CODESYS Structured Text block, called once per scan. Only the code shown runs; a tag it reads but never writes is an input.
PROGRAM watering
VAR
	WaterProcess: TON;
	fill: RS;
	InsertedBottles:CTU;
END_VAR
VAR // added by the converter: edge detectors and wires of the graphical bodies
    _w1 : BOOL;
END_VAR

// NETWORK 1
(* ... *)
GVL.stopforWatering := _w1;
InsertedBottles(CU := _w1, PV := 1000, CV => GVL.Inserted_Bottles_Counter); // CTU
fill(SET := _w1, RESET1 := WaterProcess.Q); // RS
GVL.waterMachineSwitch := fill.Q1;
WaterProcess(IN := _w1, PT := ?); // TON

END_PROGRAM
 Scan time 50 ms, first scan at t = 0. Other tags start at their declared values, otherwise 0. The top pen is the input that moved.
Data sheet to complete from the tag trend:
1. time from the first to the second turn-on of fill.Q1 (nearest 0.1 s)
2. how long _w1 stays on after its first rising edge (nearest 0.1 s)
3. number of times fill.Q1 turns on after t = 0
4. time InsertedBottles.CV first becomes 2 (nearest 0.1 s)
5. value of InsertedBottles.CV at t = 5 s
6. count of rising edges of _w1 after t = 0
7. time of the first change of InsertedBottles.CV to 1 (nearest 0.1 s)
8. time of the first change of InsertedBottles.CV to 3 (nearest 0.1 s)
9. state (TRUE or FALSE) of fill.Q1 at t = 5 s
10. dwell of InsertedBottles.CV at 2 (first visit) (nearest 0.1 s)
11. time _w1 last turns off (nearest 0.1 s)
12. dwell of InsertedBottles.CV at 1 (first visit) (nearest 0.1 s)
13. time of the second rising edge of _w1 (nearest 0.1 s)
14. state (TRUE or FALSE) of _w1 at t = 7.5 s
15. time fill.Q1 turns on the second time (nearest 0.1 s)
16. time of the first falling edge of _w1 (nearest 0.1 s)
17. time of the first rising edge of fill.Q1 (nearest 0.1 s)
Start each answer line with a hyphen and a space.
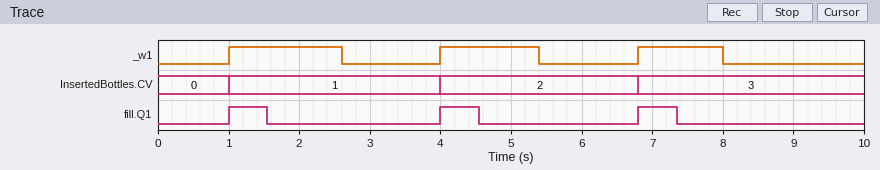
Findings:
- 3.0 s
- 1.6 s
- 3
- 4.0 s
- 2
- 3
- 1.0 s
- 6.8 s
- FALSE
- 2.8 s
- 8.0 s
- 3.0 s
- 4.0 s
- TRUE
- 4.0 s
- 2.6 s
- 1.0 s
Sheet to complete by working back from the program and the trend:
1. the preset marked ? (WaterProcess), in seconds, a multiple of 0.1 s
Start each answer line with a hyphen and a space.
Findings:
- 0.5 s
